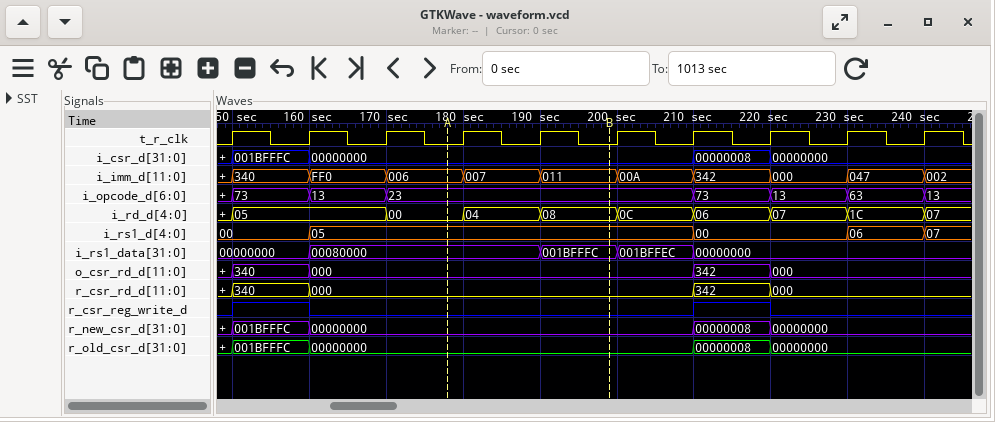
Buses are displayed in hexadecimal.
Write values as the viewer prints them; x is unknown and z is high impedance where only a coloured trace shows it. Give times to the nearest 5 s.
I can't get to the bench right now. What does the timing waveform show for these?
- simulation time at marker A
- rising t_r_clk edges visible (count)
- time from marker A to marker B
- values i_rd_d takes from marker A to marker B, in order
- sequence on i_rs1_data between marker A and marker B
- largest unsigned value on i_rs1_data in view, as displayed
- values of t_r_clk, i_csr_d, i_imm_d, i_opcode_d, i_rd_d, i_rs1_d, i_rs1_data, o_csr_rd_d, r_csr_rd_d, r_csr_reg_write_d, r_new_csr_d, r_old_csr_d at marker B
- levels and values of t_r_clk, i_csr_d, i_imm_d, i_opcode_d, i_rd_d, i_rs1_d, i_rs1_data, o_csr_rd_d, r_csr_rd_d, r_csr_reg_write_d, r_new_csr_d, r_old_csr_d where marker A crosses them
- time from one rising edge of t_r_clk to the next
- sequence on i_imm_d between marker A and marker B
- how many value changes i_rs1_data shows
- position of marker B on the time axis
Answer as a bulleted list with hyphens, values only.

- 180 s
- 10
- 20 s
- 00, 04, 08
- 00080000, 001BFFFC
- 001BFFFC
- t_r_clk=0, i_csr_d=00000000, i_imm_d=011, i_opcode_d=23, i_rd_d=08, i_rs1_d=05, i_rs1_data=001BFFFC, o_csr_rd_d=000, r_csr_rd_d=000, r_csr_reg_write_d=0, r_new_csr_d=00000000, r_old_csr_d=00000000
- t_r_clk=0, i_csr_d=00000000, i_imm_d=006, i_opcode_d=23, i_rd_d=00, i_rs1_d=05, i_rs1_data=00080000, o_csr_rd_d=000, r_csr_rd_d=000, r_csr_reg_write_d=0, r_new_csr_d=00000000, r_old_csr_d=00000000
- 10 s
- 006, 007, 011
- 4
- 200 s
